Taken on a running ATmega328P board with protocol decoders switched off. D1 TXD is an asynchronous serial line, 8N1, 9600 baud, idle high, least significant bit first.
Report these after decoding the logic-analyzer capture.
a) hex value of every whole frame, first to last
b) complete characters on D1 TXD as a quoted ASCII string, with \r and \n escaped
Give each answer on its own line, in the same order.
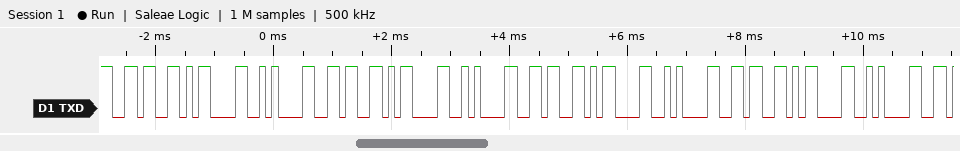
36 0D 0A 36 0D 0A 36 0D 0A 36 0D 0A
"6\r\n6\r\n6\r\n6\r\n"
